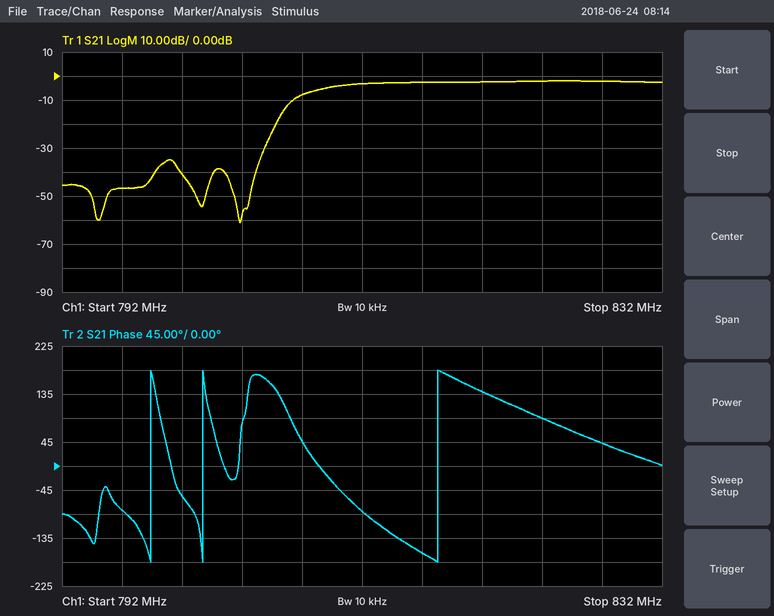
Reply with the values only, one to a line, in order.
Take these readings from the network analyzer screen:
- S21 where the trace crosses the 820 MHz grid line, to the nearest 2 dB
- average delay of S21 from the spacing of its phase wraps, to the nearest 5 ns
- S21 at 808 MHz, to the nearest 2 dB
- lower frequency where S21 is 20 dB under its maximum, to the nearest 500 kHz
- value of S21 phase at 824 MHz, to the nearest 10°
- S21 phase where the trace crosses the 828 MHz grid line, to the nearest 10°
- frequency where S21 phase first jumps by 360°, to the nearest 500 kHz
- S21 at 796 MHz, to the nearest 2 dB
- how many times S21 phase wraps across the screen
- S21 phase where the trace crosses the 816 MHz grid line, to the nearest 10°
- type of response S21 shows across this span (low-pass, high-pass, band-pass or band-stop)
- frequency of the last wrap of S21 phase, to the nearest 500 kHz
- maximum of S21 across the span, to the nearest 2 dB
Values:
-2 dB
105 ns
-8 dB
806.0 MHz
90°
40°
798.0 MHz
-46 dB
3
-160°
high-pass
817.0 MHz
-2 dB
